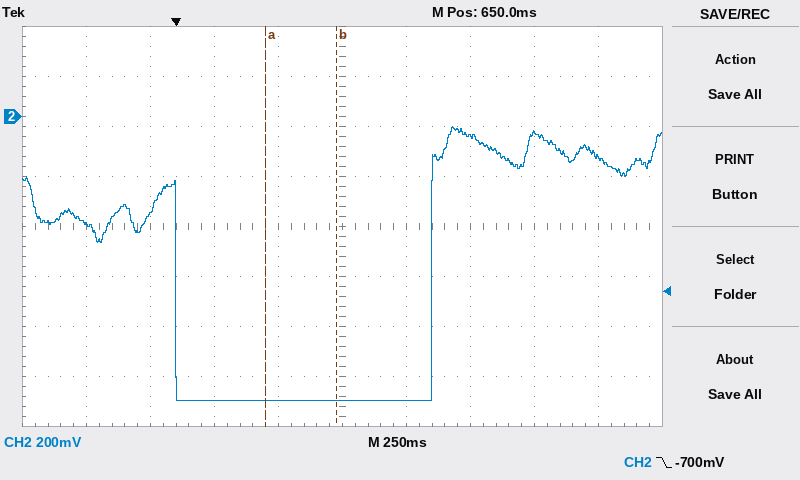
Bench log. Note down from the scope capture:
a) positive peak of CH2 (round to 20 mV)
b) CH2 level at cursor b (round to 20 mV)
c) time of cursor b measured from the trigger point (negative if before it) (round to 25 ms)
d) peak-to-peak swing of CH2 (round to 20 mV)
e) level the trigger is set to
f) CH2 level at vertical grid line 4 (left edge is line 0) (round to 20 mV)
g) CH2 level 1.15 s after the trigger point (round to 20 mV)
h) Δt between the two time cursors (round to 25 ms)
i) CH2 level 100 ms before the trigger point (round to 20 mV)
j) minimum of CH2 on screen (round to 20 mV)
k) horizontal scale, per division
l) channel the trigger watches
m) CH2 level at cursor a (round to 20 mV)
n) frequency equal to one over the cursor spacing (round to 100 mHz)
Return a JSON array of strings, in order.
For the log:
["-40 mV", "-1.14 V", "+625 ms", "1.10 V", "-700 mV", "-1.14 V", "-80 mV", "275 ms", "-380 mV", "-1.14 V", "250 ms", "CH2", "-1.14 V", "3.6 Hz"]
